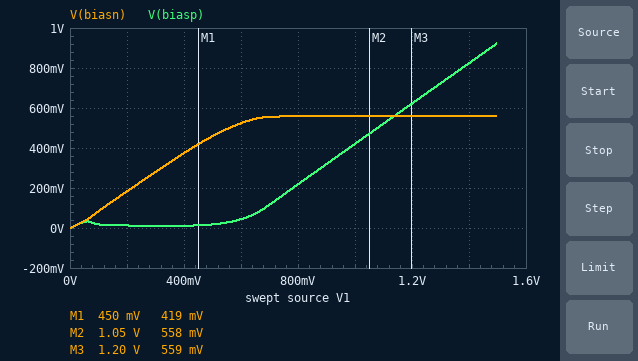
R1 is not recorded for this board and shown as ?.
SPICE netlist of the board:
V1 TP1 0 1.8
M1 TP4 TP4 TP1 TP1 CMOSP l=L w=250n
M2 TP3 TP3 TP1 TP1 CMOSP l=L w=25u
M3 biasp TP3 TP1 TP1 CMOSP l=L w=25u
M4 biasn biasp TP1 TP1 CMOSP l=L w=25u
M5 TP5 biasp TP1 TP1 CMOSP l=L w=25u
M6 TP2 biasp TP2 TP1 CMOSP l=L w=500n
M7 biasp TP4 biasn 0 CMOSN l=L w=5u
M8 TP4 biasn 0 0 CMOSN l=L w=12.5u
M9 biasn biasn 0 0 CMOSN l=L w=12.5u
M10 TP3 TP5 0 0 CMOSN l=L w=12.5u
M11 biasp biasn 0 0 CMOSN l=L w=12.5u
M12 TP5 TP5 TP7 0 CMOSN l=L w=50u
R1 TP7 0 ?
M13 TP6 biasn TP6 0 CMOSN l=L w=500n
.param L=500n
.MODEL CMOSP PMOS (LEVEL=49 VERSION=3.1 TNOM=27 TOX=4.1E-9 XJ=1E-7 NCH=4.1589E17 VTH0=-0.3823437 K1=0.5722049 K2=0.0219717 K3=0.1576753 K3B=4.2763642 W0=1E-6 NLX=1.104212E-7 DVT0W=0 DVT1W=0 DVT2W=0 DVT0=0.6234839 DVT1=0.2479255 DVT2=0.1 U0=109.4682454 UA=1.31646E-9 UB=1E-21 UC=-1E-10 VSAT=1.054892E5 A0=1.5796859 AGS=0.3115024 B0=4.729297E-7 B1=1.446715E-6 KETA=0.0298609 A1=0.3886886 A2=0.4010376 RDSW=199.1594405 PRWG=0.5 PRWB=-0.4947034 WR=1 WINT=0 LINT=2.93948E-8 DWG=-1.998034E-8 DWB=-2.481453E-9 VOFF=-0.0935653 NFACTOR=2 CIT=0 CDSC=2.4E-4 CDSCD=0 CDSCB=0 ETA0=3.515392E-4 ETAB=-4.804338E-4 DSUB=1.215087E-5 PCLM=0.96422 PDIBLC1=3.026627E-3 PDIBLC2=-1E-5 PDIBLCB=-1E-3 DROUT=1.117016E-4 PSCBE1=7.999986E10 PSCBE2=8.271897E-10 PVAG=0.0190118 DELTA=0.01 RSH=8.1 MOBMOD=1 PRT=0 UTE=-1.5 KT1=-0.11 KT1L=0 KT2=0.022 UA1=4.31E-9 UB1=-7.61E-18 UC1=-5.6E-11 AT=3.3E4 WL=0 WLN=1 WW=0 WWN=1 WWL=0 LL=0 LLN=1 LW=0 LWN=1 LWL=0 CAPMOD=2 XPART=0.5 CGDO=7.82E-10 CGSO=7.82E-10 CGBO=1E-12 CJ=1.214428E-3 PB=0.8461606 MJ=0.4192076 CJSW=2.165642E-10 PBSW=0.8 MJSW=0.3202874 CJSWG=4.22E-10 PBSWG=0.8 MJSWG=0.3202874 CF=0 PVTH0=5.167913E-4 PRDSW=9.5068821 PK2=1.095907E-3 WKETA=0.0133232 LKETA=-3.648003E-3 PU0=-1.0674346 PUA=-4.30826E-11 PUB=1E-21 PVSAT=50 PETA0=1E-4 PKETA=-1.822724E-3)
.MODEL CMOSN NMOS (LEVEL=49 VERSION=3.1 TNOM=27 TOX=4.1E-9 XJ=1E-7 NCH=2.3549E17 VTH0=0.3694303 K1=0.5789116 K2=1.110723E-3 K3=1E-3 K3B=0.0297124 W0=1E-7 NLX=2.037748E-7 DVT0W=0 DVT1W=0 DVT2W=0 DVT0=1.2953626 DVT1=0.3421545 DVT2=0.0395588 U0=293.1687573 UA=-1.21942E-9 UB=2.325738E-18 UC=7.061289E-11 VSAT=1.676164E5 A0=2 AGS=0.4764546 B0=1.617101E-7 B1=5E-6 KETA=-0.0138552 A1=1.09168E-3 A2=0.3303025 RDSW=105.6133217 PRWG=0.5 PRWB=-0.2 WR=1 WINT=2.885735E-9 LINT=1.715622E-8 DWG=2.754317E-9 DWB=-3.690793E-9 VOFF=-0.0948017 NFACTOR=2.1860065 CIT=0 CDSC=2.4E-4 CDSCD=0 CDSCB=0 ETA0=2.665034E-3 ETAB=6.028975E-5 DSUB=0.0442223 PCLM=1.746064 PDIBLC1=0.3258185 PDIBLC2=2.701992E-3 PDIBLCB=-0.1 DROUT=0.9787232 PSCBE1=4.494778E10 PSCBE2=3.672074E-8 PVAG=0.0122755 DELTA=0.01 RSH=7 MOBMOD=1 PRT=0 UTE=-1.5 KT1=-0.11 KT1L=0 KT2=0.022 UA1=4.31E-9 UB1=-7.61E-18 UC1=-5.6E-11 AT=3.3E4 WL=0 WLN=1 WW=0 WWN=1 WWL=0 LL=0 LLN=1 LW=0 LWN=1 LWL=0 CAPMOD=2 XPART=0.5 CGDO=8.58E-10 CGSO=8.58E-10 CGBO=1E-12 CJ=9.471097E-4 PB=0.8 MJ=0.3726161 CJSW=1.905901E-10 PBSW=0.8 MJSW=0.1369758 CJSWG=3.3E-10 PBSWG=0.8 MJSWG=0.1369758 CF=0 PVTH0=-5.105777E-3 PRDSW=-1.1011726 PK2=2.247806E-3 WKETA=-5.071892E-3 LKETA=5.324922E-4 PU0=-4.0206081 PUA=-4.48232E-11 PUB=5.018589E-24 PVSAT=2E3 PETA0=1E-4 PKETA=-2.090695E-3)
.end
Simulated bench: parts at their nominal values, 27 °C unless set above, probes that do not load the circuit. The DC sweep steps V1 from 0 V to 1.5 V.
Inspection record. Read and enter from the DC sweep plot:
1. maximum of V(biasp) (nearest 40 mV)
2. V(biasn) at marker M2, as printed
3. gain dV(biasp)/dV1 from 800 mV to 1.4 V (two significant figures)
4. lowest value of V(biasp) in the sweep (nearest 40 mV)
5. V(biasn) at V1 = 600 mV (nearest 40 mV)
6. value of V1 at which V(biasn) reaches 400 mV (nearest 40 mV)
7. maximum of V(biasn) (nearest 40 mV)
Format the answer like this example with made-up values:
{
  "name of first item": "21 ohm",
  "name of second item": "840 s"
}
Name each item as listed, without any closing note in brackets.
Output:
{
  "maximum of V(biasp)": "920 mV",
  "V(biasn) at marker M2, as printed": "558 mV",
  "gain dV(biasp)/dV1 from 800 mV to 1.4 V": "1.0 V/V",
  "lowest value of V(biasp) in the sweep": "0 V",
  "V(biasn) at V1 = 600 mV": "520 mV",
  "value of V1 at which V(biasn) reaches 400 mV": "440 mV",
  "maximum of V(biasn)": "560 mV"
}
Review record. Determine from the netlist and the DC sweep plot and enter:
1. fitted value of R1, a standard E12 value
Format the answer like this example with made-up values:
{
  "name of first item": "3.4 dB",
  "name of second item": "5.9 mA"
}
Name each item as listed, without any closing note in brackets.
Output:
{
  "fitted value of R1, a standard E12 value": "1.5 kΩ"
}
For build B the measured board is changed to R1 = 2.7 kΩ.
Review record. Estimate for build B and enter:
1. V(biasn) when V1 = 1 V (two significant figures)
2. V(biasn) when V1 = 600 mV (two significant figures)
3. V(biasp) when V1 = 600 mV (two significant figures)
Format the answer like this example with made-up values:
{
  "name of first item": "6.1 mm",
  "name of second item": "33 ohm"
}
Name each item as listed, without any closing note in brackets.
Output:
{
  "V(biasn) when V1 = 1 V": "520 mV",
  "V(biasn) when V1 = 600 mV": "510 mV",
  "V(biasp) when V1 = 600 mV": "68 mV"
}
